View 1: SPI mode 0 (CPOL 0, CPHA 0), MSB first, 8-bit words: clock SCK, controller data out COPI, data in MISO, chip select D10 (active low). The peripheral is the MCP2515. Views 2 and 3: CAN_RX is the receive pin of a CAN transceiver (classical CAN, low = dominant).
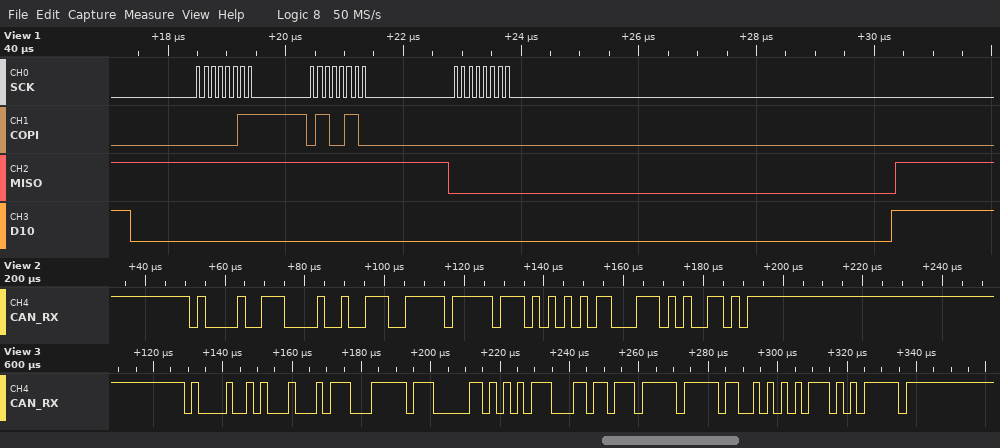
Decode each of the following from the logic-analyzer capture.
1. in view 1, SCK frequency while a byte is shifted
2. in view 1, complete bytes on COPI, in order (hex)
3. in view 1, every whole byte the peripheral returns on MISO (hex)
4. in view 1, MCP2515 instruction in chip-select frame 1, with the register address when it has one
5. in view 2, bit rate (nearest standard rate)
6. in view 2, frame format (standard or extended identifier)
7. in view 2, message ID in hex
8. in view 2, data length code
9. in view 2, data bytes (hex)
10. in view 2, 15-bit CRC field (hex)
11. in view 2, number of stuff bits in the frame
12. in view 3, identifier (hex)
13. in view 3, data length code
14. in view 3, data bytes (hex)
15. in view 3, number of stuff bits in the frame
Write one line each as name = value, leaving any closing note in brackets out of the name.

in view 1, SCK frequency while a byte is shifted = 8 MHz
in view 1, complete bytes on COPI, in order = 03 66 00
in view 1, every whole byte the peripheral returns on MISO = FF FF 00
in view 1, MCP2515 instruction in chip-select frame 1, with the register address when it has one = READ 0x66
in view 2, bit rate = 500 kbit/s
in view 2, frame format = standard
in view 2, message ID in hex = 0x427
in view 2, data length code = 4
in view 2, data bytes = 9C FF FA AB
in view 2, 15-bit CRC field = 0x0EA6
in view 2, number of stuff bits in the frame = 2
in view 3, identifier = 0x425
in view 3, data length code = 8
in view 3, data bytes = B8 FF 05 57 1B 77 FF 95
in view 3, number of stuff bits in the frame = 4
